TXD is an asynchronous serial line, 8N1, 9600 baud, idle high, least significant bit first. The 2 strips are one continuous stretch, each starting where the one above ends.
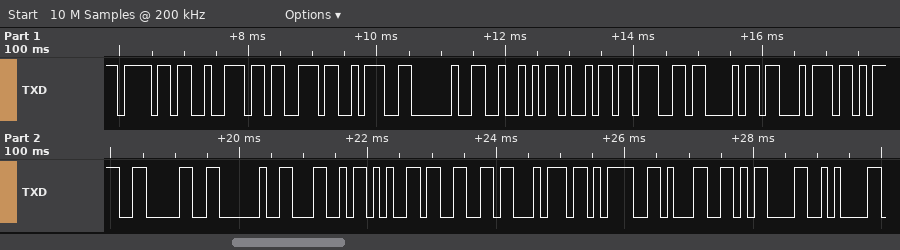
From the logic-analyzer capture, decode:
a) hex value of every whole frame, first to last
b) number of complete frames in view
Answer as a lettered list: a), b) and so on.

a) 0x6F 0x72 0x73 0x3A 0x20 0x52 0x69 0x67 0x68 0x74 0x3D 0x30 0x20 0x4C 0x65 0x66 0x74 0x3D 0x31 0x0D 0x0A
b) 21
